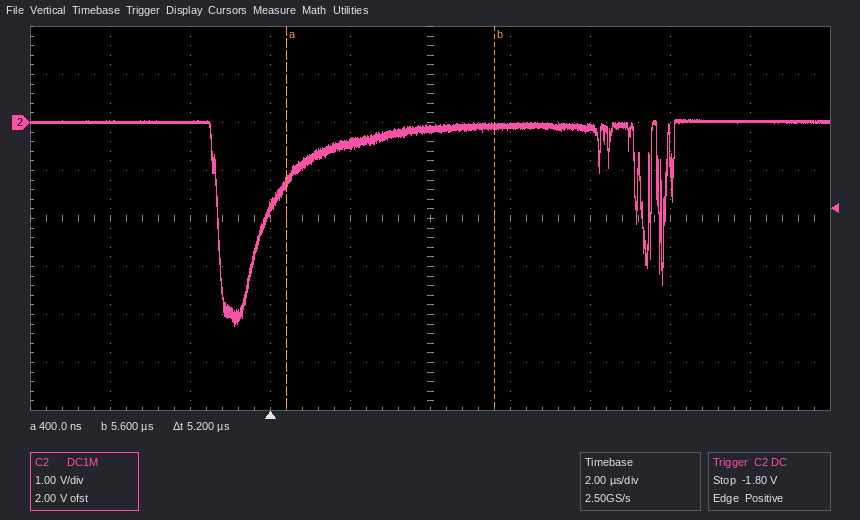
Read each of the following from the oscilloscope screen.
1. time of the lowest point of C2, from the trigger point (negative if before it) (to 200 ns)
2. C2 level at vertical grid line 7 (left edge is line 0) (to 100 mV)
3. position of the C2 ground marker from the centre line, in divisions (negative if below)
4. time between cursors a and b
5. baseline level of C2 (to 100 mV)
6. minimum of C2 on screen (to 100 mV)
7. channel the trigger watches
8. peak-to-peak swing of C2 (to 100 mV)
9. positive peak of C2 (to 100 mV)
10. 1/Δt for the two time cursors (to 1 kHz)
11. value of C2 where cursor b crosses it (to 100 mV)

-800 ns
-100 mV
+2.0 div
5.2 µs
0.0 V
-4.2 V
C2
4.3 V
100 mV
192 kHz
-100 mV
